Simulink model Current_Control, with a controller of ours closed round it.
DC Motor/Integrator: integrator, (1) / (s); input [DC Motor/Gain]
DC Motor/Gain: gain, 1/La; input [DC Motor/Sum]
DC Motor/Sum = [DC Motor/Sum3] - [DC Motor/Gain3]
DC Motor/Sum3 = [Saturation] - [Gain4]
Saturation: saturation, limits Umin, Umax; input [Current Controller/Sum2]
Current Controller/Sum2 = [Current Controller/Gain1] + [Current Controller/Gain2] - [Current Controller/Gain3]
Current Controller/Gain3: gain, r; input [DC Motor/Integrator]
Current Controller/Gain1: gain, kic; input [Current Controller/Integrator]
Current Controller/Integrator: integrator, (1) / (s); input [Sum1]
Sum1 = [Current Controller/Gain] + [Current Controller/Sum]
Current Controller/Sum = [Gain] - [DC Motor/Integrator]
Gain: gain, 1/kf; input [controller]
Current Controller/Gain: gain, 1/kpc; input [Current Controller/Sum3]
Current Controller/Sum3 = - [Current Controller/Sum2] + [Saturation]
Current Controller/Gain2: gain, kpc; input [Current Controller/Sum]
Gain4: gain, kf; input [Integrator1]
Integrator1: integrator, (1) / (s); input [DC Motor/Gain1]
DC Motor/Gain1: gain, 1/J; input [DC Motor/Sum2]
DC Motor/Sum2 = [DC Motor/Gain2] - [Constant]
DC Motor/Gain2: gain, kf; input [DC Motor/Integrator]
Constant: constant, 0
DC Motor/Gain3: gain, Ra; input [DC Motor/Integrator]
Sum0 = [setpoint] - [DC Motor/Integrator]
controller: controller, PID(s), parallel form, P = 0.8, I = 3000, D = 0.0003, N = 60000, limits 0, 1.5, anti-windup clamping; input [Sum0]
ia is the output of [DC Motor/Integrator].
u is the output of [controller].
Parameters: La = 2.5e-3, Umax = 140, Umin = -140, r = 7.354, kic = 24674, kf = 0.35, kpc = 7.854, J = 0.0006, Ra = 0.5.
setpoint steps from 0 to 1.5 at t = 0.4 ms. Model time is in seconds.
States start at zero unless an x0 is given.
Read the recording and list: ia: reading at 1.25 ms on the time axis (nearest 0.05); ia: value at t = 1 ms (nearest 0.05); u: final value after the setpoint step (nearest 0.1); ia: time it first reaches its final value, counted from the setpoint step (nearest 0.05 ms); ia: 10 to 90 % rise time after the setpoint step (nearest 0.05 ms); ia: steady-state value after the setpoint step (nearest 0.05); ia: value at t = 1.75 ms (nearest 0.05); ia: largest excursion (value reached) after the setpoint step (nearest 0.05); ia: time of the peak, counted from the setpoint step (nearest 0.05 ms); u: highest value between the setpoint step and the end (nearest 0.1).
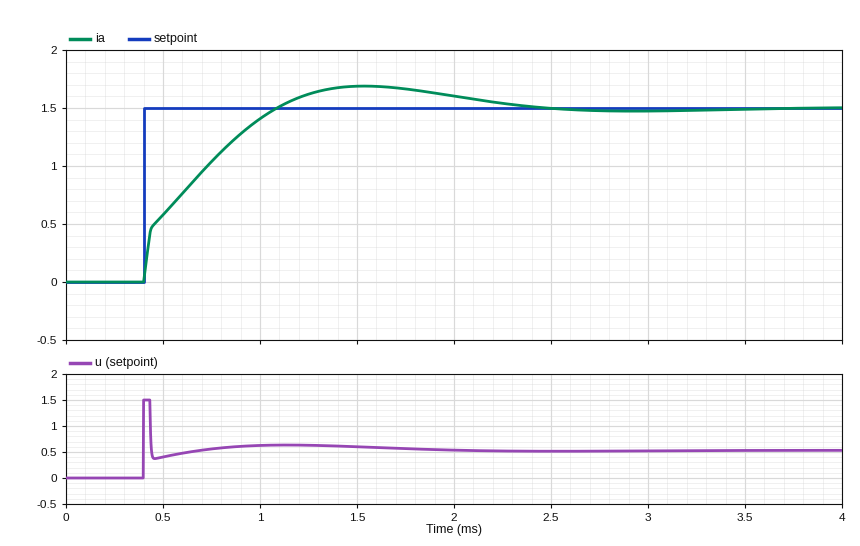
1.60
1.40
0.5
0.70 ms
0.55 ms
1.50
1.65
1.70
1.15 ms
1.5
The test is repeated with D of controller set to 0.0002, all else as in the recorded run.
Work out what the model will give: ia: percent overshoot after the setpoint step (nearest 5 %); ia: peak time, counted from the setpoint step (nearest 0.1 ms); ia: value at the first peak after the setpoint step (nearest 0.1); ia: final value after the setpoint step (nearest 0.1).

10 %
1.0 ms
1.6
1.5
